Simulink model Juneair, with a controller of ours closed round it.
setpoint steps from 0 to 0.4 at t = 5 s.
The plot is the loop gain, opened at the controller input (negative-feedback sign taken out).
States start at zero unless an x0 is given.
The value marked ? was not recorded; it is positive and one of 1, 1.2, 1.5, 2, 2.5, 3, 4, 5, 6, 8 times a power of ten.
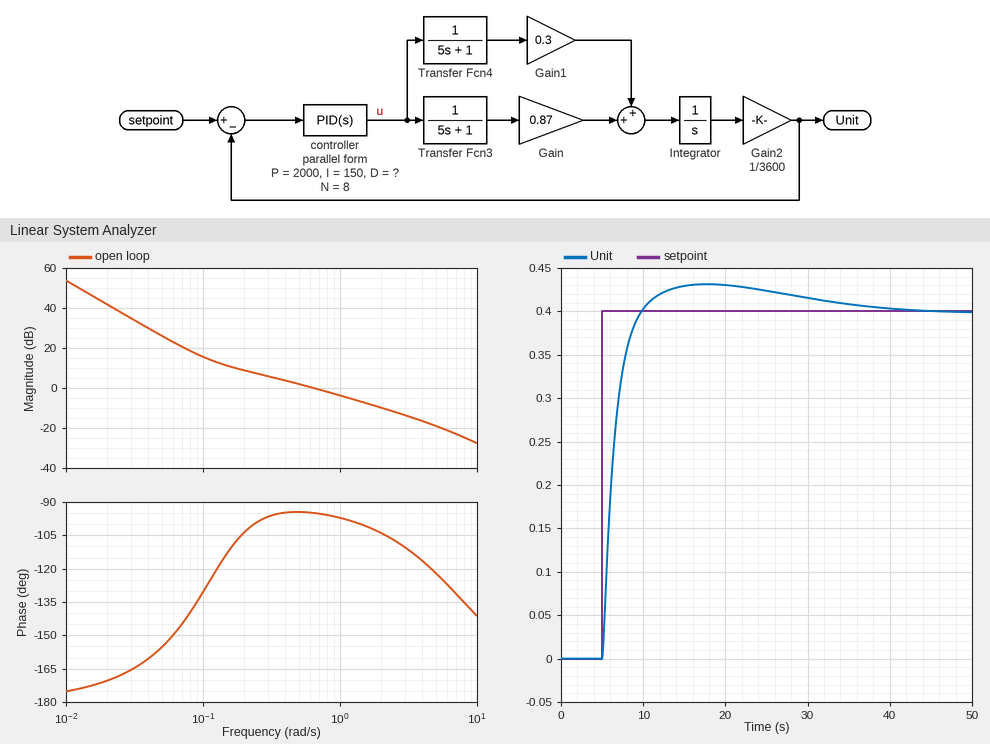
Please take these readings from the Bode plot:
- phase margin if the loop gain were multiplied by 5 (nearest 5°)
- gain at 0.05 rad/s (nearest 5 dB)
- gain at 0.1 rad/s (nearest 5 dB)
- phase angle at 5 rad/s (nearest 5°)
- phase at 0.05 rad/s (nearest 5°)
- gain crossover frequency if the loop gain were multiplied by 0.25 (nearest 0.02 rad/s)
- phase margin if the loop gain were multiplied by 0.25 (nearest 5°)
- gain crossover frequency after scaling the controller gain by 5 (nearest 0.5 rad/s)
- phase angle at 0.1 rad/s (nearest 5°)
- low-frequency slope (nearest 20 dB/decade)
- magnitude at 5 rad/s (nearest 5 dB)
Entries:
70°
25 dB
15 dB
-120°
-155°
0.14 rad/s
65°
3.0 rad/s
-130°
-40 dB/decade
-20 dB
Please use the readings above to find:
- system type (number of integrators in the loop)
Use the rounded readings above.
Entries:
2
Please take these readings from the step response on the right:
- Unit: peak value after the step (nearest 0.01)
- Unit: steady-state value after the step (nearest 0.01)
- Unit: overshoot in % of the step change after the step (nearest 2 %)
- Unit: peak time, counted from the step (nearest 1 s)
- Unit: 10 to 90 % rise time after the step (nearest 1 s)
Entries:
0.43
0.40
8 %
13 s
3 s
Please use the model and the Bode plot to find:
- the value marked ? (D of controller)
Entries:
10000
